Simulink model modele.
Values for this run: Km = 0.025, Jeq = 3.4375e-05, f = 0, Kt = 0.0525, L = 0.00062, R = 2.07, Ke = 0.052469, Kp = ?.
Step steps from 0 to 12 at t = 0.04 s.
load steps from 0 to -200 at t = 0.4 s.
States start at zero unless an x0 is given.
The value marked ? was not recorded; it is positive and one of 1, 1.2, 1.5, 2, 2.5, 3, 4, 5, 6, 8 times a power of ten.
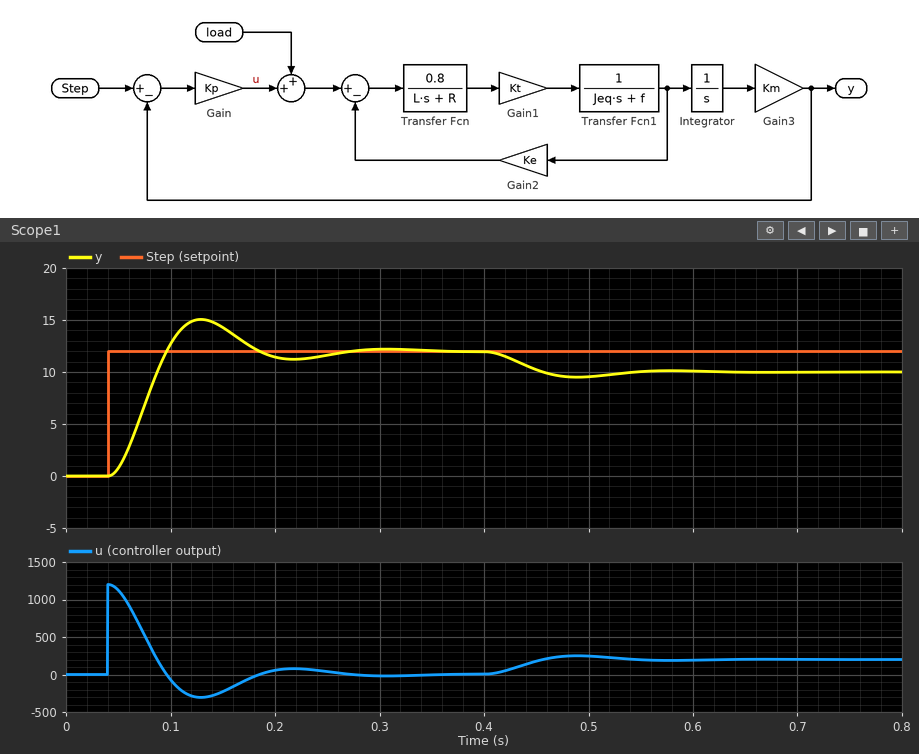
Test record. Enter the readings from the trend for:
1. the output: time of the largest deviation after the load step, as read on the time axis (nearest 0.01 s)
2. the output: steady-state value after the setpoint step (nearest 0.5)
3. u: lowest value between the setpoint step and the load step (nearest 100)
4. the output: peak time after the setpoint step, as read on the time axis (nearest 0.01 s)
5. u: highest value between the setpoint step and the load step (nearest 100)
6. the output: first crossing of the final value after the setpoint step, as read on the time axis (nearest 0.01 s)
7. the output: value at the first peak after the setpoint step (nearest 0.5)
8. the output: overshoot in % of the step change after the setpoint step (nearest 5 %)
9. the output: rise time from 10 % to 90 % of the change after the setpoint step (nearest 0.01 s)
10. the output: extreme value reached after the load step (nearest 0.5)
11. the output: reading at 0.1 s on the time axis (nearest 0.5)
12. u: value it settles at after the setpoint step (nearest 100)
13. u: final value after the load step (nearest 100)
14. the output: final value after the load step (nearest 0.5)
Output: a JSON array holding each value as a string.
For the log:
["0.49 s", "12.0", "-300", "0.13 s", "1200", "0.10 s", "15.0", "25 %", "0.04 s", "9.5", "12.5", "0", "200", "10.0"]
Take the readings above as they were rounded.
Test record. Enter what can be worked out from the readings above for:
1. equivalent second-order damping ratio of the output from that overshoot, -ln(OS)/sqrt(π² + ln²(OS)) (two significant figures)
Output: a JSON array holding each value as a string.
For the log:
["0.40"]
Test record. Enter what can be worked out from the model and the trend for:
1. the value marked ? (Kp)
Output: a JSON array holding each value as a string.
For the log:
["100"]
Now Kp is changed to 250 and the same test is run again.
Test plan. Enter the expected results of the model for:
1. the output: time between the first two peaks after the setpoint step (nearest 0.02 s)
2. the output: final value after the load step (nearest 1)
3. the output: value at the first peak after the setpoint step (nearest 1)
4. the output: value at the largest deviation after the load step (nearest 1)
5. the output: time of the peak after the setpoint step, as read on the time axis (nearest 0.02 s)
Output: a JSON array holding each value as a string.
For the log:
["0.10 s", "11", "17", "11", "0.10 s"]
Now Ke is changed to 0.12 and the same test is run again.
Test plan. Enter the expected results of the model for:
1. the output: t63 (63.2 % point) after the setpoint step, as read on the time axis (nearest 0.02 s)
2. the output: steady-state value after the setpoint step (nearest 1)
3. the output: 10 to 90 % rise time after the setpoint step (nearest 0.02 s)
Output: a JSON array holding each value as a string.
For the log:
["0.10 s", "12", "0.08 s"]
